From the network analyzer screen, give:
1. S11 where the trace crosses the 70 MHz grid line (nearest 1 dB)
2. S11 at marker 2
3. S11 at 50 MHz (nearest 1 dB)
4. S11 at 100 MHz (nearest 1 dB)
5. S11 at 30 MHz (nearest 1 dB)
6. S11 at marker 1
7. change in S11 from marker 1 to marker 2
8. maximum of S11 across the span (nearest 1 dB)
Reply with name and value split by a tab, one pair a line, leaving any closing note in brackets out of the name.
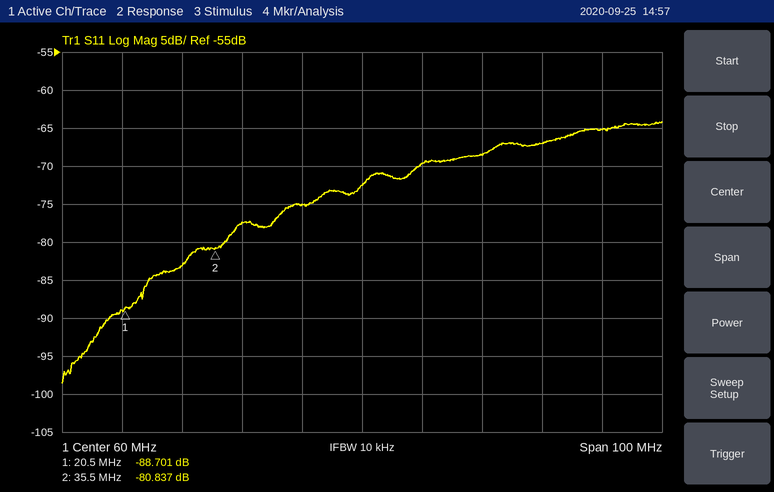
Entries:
S11 where the trace crosses the 70 MHz grid line	-70 dB
S11 at marker 2	-80.837 dB
S11 at 50 MHz	-75 dB
S11 at 100 MHz	-65 dB
S11 at 30 MHz	-83 dB
S11 at marker 1	-88.701 dB
change in S11 from marker 1 to marker 2	7.864 dB
maximum of S11 across the span	-64 dB
